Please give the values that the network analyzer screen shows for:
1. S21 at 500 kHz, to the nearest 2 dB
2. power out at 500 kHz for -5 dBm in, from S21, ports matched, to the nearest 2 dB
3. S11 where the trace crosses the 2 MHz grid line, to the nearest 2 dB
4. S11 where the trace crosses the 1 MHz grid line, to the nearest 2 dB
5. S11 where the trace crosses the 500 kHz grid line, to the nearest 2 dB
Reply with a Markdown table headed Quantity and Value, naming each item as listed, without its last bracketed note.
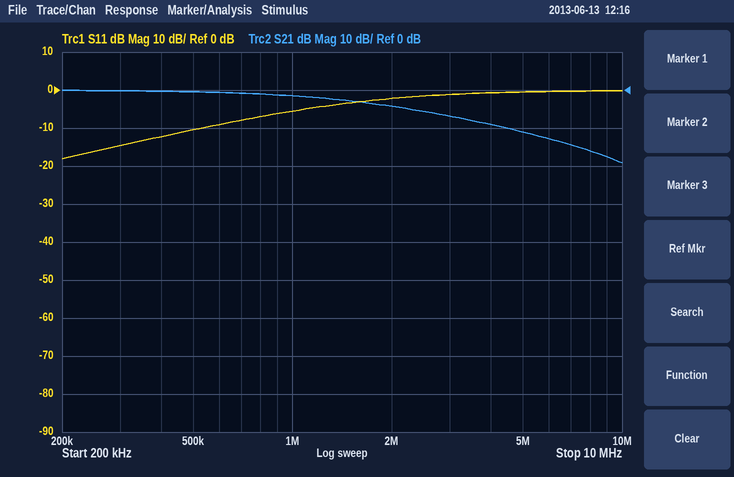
| Quantity | Value |
|---|---|
| S21 at 500 kHz, to the nearest 2 dB | 0 dB |
| power out at 500 kHz for -5 dBm in, from S21, ports matched, to the nearest 2 dB | -6 dBm |
| S11 where the trace crosses the 2 MHz grid line, to the nearest 2 dB | -2 dB |
| S11 where the trace crosses the 1 MHz grid line, to the nearest 2 dB | -6 dB |
| S11 where the trace crosses the 500 kHz grid line, to the nearest 2 dB | -10 dB |
